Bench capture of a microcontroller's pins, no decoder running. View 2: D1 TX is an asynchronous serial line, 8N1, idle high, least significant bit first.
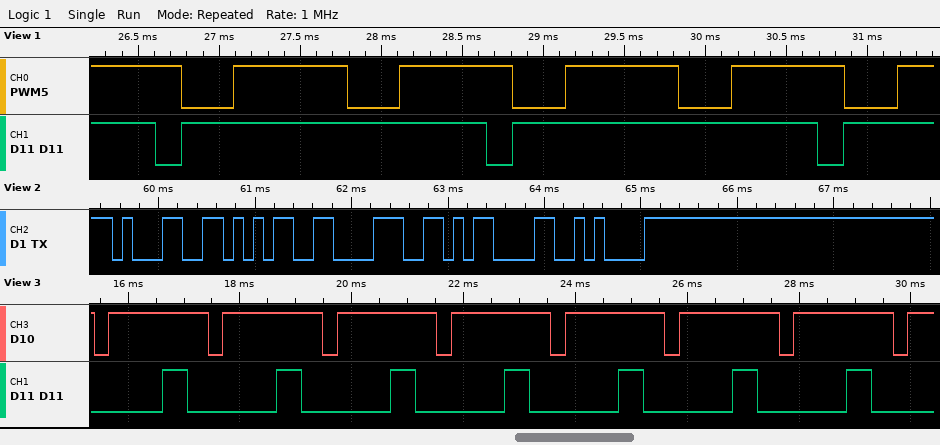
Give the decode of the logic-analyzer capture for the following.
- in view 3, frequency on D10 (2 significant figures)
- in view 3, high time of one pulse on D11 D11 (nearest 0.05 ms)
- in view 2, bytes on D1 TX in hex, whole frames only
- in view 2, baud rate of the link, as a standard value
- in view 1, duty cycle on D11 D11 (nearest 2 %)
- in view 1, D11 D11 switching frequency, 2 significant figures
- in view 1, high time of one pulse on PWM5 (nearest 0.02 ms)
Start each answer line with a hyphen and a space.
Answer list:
- 490 Hz
- 0.45 ms
- 31 35 38 0D 0A
- 9600 baud
- 92 %
- 490 Hz
- 0.70 ms
